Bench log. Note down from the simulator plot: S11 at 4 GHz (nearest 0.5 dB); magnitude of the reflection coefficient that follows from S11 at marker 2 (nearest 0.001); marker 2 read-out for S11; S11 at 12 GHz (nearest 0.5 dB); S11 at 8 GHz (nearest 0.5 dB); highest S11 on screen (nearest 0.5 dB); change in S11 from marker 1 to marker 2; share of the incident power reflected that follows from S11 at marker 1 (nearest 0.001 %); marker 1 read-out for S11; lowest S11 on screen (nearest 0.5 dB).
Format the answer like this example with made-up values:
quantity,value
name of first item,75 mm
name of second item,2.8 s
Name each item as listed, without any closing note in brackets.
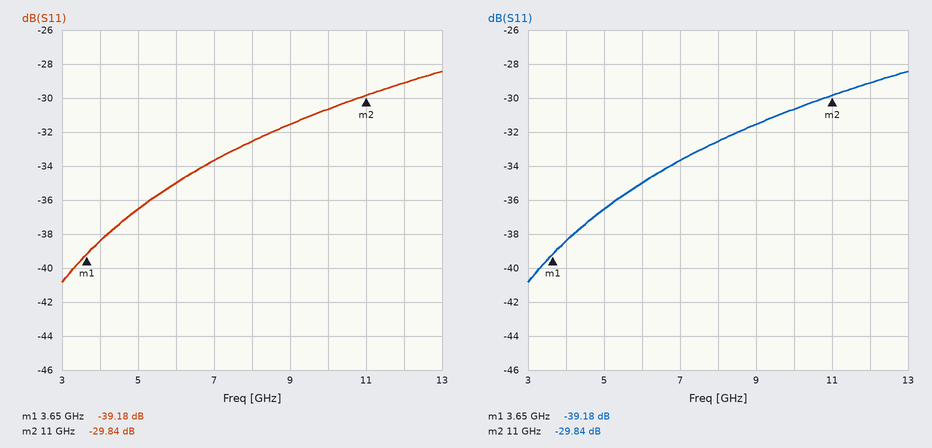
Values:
quantity,value
S11 at 4 GHz,-38.5 dB
magnitude of the reflection coefficient that follows from S11 at marker 2,0.032
marker 2 read-out for S11,-29.84 dB
S11 at 12 GHz,-29.0 dB
S11 at 8 GHz,-32.5 dB
highest S11 on screen,-28.5 dB
change in S11 from marker 1 to marker 2,9.34 dB
share of the incident power reflected that follows from S11 at marker 1,0.012 %
marker 1 read-out for S11,-39.18 dB
lowest S11 on screen,-41.0 dB
